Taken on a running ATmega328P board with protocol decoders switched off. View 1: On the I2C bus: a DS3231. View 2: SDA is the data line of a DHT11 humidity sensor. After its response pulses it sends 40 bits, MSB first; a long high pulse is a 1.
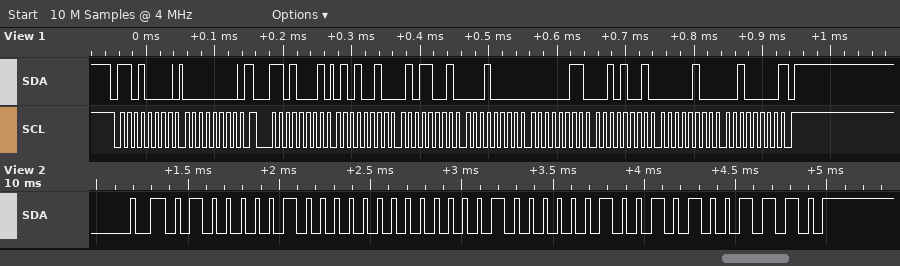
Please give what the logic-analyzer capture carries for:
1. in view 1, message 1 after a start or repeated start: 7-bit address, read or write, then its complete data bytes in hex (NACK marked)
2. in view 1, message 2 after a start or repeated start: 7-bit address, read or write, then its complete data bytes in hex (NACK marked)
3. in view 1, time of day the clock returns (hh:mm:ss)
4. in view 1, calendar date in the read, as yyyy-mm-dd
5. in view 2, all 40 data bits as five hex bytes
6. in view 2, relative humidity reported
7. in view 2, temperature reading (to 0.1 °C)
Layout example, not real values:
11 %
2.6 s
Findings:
0x68 write: 00
0x68 read: 52 59 10 03 29 04 20 NACK
10:59:52
2020-04-29
41 00 04 09 4E
65 %
4.9 °C
